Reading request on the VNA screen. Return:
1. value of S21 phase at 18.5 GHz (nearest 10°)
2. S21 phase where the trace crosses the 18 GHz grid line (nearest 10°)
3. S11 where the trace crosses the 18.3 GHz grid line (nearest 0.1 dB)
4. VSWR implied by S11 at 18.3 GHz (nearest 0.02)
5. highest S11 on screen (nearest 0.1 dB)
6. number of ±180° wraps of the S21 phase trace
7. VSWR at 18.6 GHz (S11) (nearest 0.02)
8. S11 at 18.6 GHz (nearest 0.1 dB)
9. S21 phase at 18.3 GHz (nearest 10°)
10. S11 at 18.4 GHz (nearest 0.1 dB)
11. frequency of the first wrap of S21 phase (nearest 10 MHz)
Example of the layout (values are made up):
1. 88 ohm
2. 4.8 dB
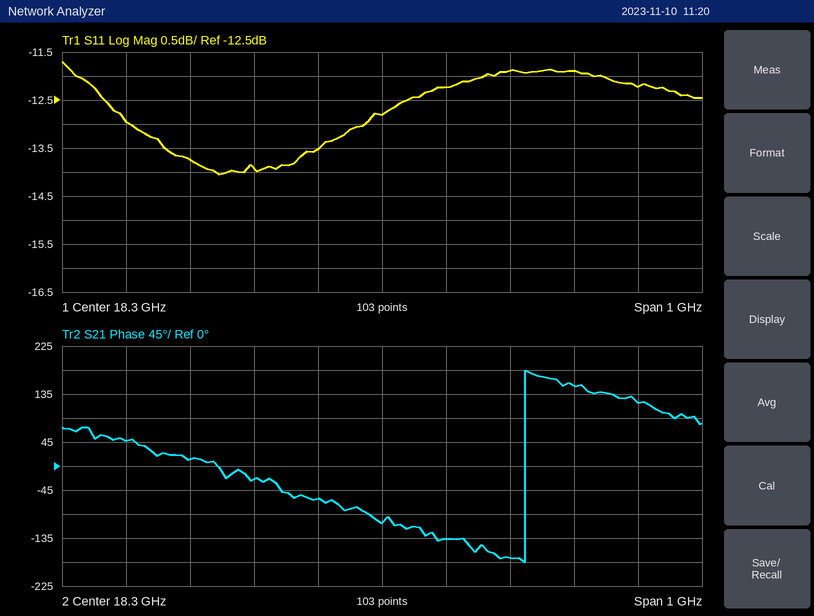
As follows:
1. -170°
2. 10°
3. -12.8 dB
4. 1.60
5. -11.7 dB
6. 1
7. 1.68
8. -11.9 dB
9. -110°
10. -12.2 dB
11. 18.52 GHz
